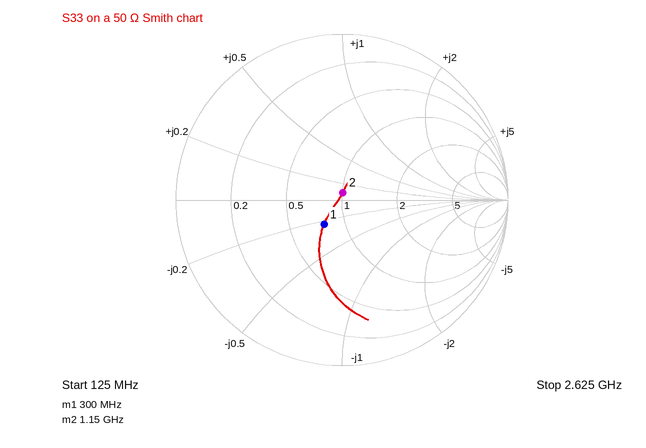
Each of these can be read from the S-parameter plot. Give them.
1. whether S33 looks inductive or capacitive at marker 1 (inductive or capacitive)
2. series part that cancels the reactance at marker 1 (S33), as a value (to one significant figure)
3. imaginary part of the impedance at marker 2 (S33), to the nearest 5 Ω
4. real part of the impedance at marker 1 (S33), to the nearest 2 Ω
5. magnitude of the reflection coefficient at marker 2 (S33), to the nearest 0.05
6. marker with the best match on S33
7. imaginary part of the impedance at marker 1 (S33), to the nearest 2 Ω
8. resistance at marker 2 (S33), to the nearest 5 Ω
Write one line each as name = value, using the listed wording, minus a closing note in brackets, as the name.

whether S33 looks inductive or capacitive at marker 1 = capacitive
series part that cancels the reactance at marker 1 (S33), as a value = 6 nH
imaginary part of the impedance at marker 2 (S33), to the nearest 5 Ω = +5 Ω
real part of the impedance at marker 1 (S33), to the nearest 2 Ω = 38 Ω
magnitude of the reflection coefficient at marker 2 (S33), to the nearest 0.05 = 0.05
marker with the best match on S33 = marker 2
imaginary part of the impedance at marker 1 (S33), to the nearest 2 Ω = -12 Ω
resistance at marker 2 (S33), to the nearest 5 Ω = 50 Ω
